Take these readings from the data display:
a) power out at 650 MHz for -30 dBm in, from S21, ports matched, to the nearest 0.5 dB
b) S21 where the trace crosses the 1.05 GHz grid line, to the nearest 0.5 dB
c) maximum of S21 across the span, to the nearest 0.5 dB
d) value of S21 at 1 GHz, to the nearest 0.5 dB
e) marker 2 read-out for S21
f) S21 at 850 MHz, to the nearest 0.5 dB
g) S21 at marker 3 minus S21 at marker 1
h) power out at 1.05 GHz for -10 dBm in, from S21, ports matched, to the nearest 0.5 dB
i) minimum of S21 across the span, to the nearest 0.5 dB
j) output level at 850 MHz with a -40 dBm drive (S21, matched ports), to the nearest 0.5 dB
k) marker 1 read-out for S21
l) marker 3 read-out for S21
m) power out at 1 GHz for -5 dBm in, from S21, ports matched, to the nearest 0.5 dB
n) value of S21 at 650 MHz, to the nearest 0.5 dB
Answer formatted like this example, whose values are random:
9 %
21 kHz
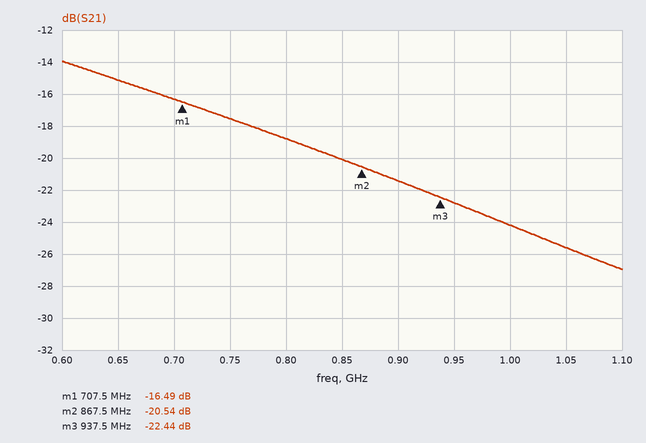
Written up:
-45.0 dBm
-25.5 dB
-14.0 dB
-24.0 dB
-20.54 dB
-20.0 dB
-5.95 dB
-35.5 dBm
-27.0 dB
-60.0 dBm
-16.49 dB
-22.44 dB
-29.0 dBm
-15.0 dB
